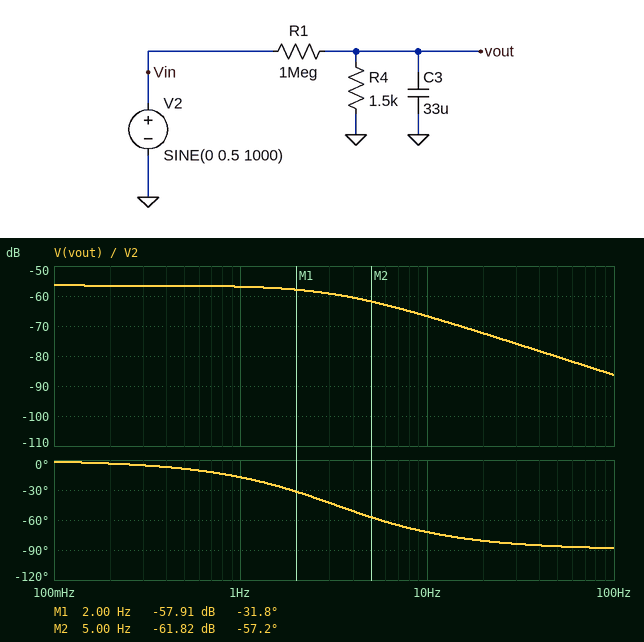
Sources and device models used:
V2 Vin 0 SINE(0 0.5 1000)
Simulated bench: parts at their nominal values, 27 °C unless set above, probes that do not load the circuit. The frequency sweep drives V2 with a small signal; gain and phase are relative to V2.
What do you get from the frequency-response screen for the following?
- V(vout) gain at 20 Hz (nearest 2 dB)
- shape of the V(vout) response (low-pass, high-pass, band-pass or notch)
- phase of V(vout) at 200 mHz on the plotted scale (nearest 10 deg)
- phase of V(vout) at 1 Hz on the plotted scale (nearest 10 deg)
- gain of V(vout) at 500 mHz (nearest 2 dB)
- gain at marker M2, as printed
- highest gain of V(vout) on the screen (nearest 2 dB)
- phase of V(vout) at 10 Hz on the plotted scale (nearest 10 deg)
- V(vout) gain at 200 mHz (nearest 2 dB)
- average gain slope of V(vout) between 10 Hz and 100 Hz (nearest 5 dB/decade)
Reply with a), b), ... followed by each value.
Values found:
a) -72 dB
b) low-pass
c) 0 deg
d) -20 deg
e) -56 dB
f) -61.82 dB
g) -56 dB
h) -70 deg
i) -56 dB
j) -20 dB/decade
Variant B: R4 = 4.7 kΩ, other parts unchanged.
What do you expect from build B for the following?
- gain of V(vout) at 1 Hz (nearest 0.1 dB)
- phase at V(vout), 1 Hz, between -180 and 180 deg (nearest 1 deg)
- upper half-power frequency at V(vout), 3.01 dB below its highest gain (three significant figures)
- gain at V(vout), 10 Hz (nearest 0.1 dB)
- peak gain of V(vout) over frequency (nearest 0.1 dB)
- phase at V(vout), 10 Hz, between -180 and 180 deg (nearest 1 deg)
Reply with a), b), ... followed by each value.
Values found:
a) -49.5 dB
b) -44 deg
c) 1.03 Hz
d) -66.4 dB
e) -46.6 dB
f) -84 deg
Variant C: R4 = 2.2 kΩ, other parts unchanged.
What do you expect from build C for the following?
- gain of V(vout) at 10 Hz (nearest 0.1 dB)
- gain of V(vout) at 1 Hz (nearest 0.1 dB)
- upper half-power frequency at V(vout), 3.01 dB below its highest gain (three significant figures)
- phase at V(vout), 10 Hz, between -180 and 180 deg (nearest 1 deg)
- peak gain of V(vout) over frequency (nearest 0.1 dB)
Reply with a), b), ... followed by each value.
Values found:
a) -66.5 dB
b) -54.0 dB
c) 2.20 Hz
d) -78 deg
e) -53.2 dB
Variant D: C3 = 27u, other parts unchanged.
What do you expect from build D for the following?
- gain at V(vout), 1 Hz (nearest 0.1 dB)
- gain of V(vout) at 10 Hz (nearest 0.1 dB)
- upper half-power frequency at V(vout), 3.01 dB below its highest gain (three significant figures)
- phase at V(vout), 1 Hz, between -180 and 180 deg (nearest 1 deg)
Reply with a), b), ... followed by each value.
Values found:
a) -56.8 dB
b) -65.2 dB
c) 3.94 Hz
d) -14 deg
